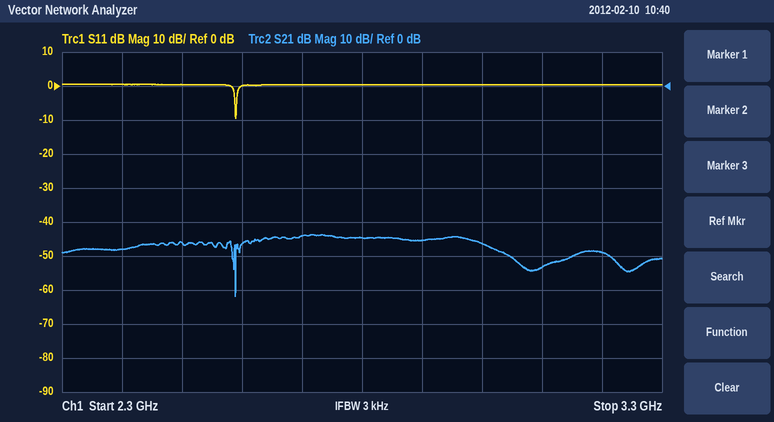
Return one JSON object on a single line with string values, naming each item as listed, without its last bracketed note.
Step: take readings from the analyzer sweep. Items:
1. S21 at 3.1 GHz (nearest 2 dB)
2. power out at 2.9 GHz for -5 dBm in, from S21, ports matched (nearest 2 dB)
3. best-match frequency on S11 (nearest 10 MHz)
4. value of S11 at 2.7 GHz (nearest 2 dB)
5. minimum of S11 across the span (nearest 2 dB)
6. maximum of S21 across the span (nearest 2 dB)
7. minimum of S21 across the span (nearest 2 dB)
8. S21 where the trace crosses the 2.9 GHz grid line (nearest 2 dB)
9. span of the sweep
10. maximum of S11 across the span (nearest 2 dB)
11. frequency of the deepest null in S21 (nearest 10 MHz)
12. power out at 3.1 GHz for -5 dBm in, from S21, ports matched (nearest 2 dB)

{"S21 at 3.1 GHz": "-54 dB", "power out at 2.9 GHz for -5 dBm in, from S21, ports matched": "-50 dBm", "best-match frequency on S11": "2.59 GHz", "value of S11 at 2.7 GHz": "0 dB", "minimum of S11 across the span": "-10 dB", "maximum of S21 across the span": "-44 dB", "minimum of S21 across the span": "-62 dB", "S21 where the trace crosses the 2.9 GHz grid line": "-46 dB", "span of the sweep": "1 GHz", "maximum of S11 across the span": "0 dB", "frequency of the deepest null in S21": "2.59 GHz", "power out at 3.1 GHz for -5 dBm in, from S21, ports matched": "-58 dBm"}
